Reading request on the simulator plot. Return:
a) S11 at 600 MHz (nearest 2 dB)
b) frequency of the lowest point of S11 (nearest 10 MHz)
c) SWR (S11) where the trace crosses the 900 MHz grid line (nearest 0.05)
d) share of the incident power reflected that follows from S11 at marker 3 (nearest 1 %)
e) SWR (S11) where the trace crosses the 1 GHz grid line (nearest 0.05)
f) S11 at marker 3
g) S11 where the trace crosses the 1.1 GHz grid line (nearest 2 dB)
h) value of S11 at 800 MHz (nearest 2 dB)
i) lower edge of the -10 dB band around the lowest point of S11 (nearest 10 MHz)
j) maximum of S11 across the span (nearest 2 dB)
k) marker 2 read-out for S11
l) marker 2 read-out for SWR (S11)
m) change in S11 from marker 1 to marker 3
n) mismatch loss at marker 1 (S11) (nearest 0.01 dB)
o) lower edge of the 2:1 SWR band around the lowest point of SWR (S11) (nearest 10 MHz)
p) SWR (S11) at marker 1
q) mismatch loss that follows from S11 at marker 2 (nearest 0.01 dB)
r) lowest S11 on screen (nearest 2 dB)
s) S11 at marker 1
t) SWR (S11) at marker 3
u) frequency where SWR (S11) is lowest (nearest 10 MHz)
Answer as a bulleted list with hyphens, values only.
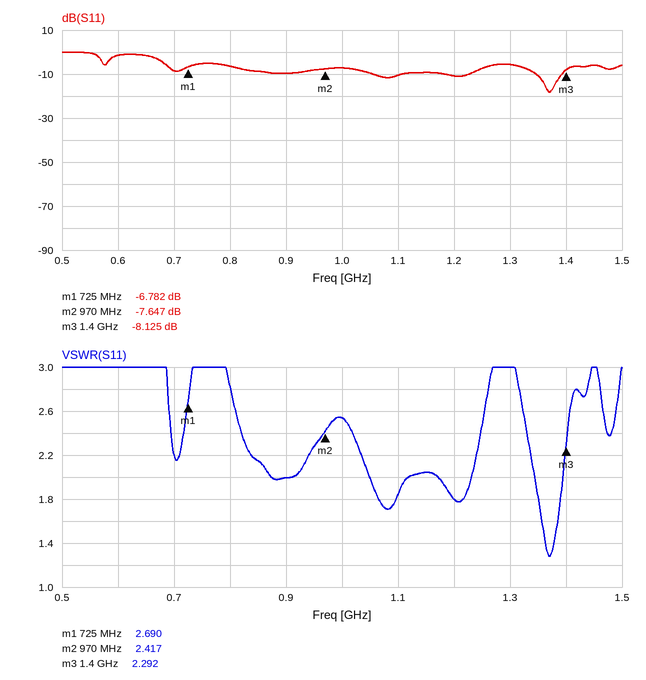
- -2 dB
- 1.37 GHz
- 2.00
- 15 %
- 2.55
- -8.125 dB
- -10 dB
- -6 dB
- 1.35 GHz
- 0 dB
- -7.647 dB
- 2.417
- -1.343 dB
- 1.02 dB
- 1.34 GHz
- 2.690
- 0.82 dB
- -18 dB
- -6.782 dB
- 2.292
- 1.37 GHz
